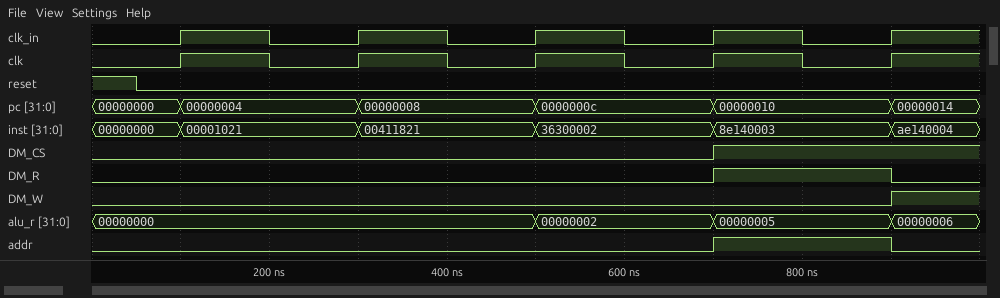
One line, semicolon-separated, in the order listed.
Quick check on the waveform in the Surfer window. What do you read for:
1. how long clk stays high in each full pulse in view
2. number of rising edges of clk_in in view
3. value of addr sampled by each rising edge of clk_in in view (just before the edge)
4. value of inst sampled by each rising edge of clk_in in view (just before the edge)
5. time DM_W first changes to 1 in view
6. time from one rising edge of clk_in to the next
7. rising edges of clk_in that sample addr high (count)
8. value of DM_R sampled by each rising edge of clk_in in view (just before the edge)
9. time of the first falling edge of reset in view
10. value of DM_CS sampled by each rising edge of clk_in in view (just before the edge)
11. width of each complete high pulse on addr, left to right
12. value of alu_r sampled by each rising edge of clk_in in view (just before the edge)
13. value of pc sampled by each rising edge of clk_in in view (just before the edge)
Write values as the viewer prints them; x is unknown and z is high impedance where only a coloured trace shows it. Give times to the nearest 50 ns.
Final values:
100 ns, 100 ns, 100 ns, 100 ns; 5; 0 0 0 0 1; 00000000, 00001021, 00411821, 36300002, 8e140003; 900 ns; 200 ns; 1; 0 0 0 0 1; 50 ns; 0 0 0 0 1; 200 ns; 00000000, 00000000, 00000000, 00000002, 00000005; 00000000, 00000004, 00000008, 0000000c, 00000010
